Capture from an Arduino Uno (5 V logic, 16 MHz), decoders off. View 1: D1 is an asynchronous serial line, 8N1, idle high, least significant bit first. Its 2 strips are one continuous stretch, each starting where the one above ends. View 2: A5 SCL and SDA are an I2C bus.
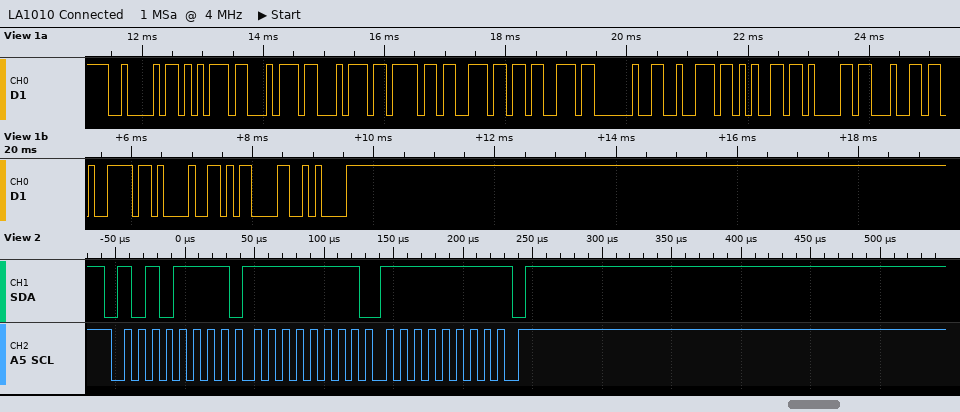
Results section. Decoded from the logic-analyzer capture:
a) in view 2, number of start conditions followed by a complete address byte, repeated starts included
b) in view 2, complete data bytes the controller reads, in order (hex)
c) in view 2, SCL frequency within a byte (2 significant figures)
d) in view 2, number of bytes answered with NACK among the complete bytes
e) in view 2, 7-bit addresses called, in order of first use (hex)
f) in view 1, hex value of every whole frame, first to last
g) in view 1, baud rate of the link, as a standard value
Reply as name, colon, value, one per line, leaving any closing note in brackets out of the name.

in view 2, number of start conditions followed by a complete address byte, repeated starts included: 1
in view 2, complete data bytes the controller reads, in order: FF FF
in view 2, SCL frequency within a byte: 100 kHz
in view 2, number of bytes answered with NACK among the complete bytes: 1
in view 2, 7-bit addresses called, in order of first use: 0x57
in view 1, hex value of every whole frame, first to last: 42 75 74 74 6F 6E 73 20 72 65 61 64 79 21 0D 0A
in view 1, baud rate of the link, as a standard value: 9600 baud
